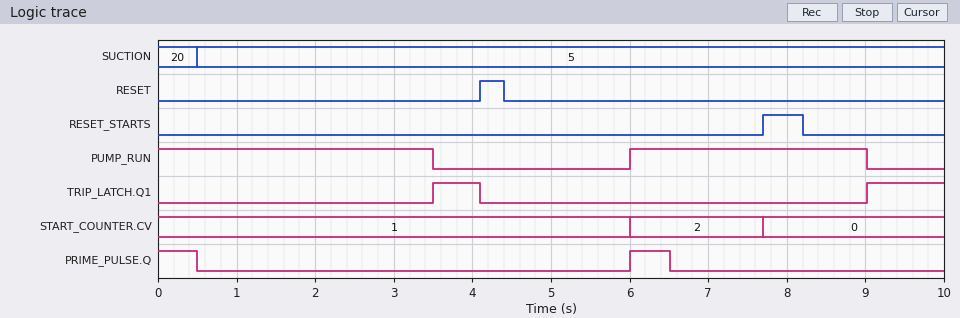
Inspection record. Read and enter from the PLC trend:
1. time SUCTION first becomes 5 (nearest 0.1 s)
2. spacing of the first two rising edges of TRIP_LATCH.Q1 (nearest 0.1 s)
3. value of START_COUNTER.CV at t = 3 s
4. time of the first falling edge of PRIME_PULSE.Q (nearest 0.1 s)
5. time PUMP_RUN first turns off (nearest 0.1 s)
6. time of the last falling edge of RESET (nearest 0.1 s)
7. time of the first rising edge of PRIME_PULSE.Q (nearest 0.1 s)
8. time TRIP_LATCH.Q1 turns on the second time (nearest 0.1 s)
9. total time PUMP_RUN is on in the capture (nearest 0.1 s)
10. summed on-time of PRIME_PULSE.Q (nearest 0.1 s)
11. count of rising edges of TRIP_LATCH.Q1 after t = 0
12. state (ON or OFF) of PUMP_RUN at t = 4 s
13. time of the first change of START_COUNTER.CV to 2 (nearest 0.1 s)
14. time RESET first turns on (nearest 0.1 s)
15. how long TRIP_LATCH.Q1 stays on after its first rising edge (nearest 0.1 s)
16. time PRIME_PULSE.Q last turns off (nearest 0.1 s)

0.5 s
5.5 s
1
0.5 s
3.5 s
4.4 s
6.0 s
9.0 s
6.5 s
1.0 s
2
OFF
6.0 s
4.1 s
0.6 s
6.5 s
